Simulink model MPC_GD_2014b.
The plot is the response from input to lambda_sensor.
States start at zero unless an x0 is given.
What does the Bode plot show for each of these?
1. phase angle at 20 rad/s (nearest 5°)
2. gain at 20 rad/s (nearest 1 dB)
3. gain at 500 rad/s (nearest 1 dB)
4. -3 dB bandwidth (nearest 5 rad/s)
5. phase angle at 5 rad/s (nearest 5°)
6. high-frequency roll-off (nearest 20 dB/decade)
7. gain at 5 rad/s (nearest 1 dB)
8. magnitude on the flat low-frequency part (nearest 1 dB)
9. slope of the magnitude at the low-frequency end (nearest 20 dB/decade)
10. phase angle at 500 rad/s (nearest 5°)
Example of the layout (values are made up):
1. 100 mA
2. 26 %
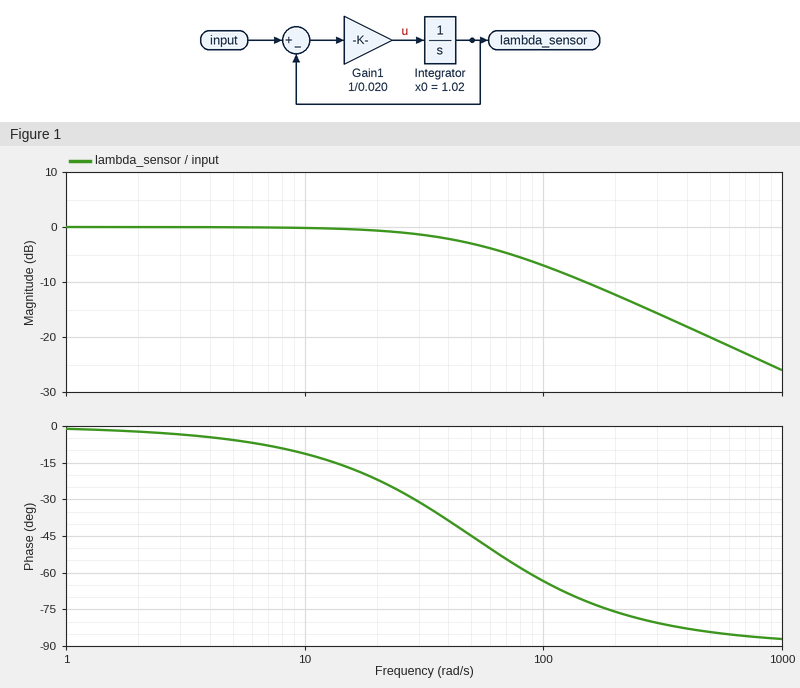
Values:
1. -20°
2. -1 dB
3. -20 dB
4. 50 rad/s
5. -5°
6. -20 dB/decade
7. 0 dB
8. 0 dB
9. 0 dB/decade
10. -85°
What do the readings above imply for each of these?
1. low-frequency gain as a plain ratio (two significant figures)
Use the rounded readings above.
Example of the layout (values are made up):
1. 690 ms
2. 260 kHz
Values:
1. 1.0
